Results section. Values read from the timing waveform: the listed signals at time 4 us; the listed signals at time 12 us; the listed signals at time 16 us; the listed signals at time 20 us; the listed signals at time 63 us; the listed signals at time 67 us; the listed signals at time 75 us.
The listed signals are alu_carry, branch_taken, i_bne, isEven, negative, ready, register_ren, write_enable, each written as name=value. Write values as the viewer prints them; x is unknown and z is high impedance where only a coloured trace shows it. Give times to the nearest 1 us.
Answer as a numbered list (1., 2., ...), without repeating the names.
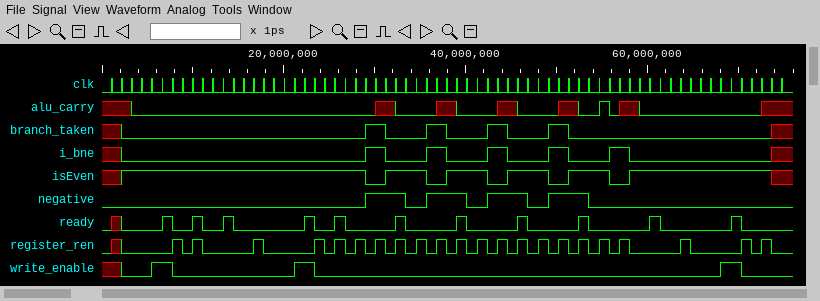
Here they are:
1. alu_carry=0, branch_taken=0, i_bne=0, isEven=1, negative=0, ready=0, register_ren=0, write_enable=0
2. alu_carry=0, branch_taken=0, i_bne=0, isEven=1, negative=0, ready=0, register_ren=0, write_enable=0
3. alu_carry=0, branch_taken=0, i_bne=0, isEven=1, negative=0, ready=0, register_ren=0, write_enable=0
4. alu_carry=0, branch_taken=0, i_bne=0, isEven=1, negative=0, ready=0, register_ren=0, write_enable=0
5. alu_carry=0, branch_taken=0, i_bne=0, isEven=1, negative=0, ready=0, register_ren=0, write_enable=0
6. alu_carry=0, branch_taken=0, i_bne=0, isEven=1, negative=0, ready=0, register_ren=0, write_enable=0
7. alu_carry=x, branch_taken=x, i_bne=x, isEven=x, negative=0, ready=0, register_ren=0, write_enable=0
